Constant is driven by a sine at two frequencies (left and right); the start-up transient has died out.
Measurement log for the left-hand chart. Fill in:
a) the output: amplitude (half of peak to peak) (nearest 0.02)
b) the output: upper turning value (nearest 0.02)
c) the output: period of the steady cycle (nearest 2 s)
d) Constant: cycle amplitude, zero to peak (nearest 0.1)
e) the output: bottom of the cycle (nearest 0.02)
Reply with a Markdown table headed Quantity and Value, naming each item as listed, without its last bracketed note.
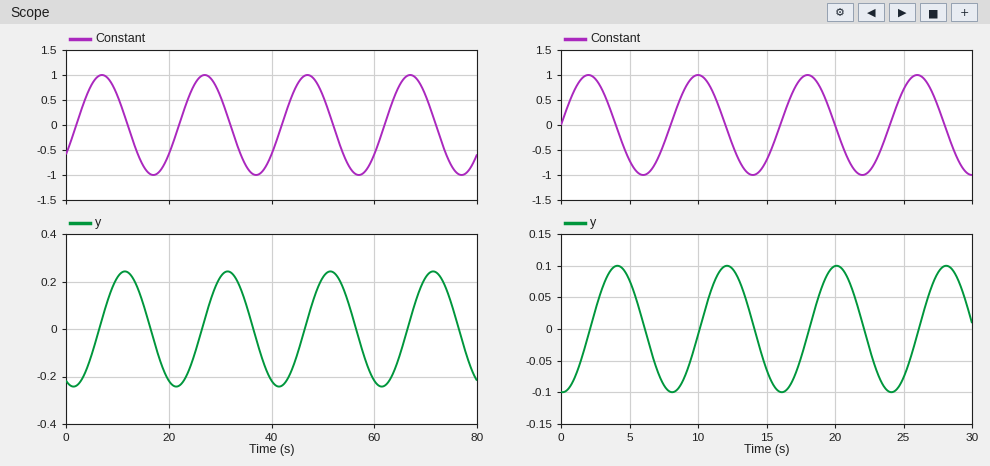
| Quantity | Value |
|---|---|
| the output: amplitude (half of peak to peak) | 0.24 |
| the output: upper turning value | 0.24 |
| the output: period of the steady cycle | 20 s |
| Constant: cycle amplitude, zero to peak | 1.0 |
| the output: bottom of the cycle | -0.24 |
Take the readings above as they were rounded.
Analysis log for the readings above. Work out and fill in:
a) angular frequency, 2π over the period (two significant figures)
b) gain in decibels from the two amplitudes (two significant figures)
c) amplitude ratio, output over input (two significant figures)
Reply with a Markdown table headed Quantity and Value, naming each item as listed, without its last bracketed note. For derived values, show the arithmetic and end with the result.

| Quantity | Value |
|---|---|
| angular frequency, 2π over the period | 2π / 20 = 0.31 rad/s |
| gain in decibels from the two amplitudes | 20 log10(0.24 / 1) = -12 dB |
| amplitude ratio, output over input | 0.24 / 1 = 0.24 |
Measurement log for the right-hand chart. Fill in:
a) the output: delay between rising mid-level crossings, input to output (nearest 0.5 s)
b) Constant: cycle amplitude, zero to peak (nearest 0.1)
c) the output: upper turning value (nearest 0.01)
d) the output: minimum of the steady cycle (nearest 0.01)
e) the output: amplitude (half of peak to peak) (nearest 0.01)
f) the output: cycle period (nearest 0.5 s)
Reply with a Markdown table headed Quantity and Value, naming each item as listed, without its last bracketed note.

| Quantity | Value |
|---|---|
| the output: delay between rising mid-level crossings, input to output | 2.0 s |
| Constant: cycle amplitude, zero to peak | 1.0 |
| the output: upper turning value | 0.10 |
| the output: minimum of the steady cycle | -0.10 |
| the output: amplitude (half of peak to peak) | 0.10 |
| the output: cycle period | 8.0 s |
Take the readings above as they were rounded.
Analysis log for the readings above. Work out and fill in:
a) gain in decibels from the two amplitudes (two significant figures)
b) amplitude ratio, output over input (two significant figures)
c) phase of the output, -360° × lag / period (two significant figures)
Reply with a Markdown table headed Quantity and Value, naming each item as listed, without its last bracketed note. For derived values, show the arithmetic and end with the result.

| Quantity | Value |
|---|---|
| gain in decibels from the two amplitudes | 20 log10(0.1 / 1) = -20 dB |
| amplitude ratio, output over input | 0.1 / 1 = 0.10 |
| phase of the output, -360° × lag / period | -360 × 2 / 8 = -90° |
